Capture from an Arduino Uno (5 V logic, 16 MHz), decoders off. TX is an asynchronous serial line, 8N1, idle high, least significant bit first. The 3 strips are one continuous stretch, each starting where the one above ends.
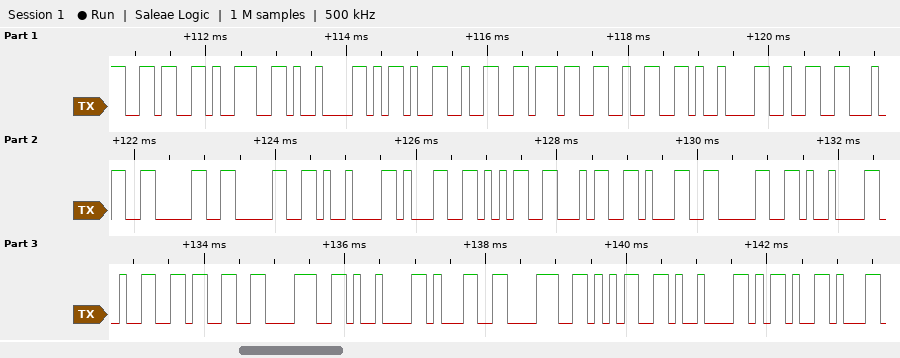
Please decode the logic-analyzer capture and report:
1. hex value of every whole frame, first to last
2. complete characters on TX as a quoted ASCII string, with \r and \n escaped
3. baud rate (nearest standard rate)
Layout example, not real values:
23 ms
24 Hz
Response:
36 39 09 2D 32 37 32 09 32 34 30 30 09 31 35 34 31 30 09 32 33 38 09 31 38 35 09 2D
"69\t-272\t2400\t15410\t238\t185\t-"
9600 baud
